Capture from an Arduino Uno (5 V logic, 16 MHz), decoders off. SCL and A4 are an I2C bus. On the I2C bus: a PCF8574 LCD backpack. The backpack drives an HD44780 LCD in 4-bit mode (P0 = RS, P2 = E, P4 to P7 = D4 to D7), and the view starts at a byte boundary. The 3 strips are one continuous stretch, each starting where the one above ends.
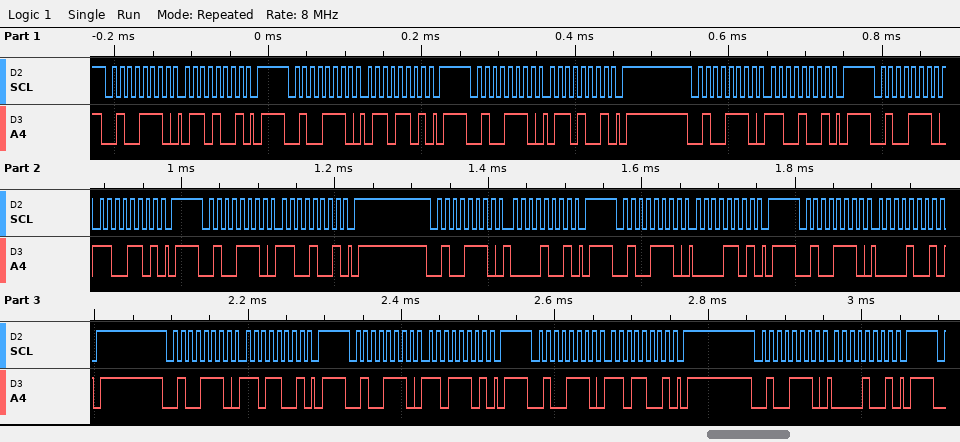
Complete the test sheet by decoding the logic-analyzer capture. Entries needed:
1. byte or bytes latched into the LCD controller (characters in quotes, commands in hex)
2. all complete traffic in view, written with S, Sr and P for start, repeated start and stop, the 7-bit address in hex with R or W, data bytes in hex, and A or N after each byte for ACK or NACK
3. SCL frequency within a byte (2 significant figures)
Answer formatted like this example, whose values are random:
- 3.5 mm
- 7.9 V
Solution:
- 'l' data 0x0D
- S 27W A 69 A P S 27W A 6D A P S 27W A 69 A P S 27W A C9 A P S 27W A CD A P S 27W A C9 A P S 27W A 09 A P S 27W A 0D A P S 27W A 09 A P S 27W A D9 A P S 27W A DD A P S 27W A D9 A P S 27W A 09 A P
- 100 kHz
